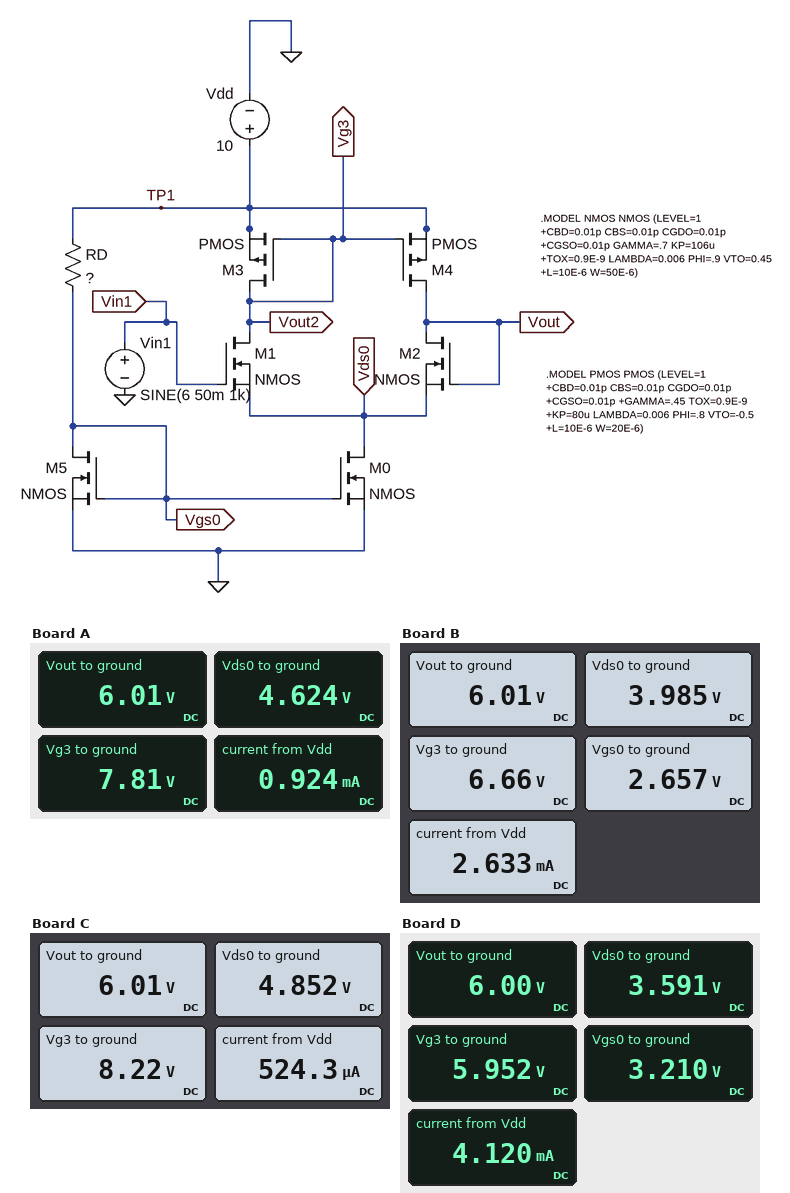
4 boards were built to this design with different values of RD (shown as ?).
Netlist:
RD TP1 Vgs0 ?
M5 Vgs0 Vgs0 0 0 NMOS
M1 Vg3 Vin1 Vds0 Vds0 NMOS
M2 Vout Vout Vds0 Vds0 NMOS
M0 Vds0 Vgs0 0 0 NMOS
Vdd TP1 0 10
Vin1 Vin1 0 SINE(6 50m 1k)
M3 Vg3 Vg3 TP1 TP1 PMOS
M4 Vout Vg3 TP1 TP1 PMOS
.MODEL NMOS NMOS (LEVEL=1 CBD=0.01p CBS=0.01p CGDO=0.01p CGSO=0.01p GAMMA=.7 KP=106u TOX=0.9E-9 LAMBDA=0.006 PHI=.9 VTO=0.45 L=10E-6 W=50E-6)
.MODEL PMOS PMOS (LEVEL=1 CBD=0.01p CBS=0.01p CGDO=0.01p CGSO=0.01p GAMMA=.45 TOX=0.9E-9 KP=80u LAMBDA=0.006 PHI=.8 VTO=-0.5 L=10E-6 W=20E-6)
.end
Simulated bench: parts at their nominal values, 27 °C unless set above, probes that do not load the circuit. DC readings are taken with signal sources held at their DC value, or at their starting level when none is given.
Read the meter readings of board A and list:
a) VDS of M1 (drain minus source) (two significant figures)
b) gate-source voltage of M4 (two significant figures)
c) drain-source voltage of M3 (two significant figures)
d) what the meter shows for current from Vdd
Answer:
3.2 V
-2.2 V
-2.2 V
0.924 mA
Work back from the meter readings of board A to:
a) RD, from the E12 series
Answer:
18 kΩ
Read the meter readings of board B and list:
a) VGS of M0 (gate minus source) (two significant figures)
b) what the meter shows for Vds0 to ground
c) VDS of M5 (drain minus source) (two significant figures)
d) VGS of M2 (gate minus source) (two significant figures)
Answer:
2.7 V
3.985 V
2.7 V
2.0 V
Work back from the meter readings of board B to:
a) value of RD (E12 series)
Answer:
5.6 kΩ
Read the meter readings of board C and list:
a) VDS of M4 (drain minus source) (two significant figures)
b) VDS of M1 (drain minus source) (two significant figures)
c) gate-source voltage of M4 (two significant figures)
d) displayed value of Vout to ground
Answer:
-4.0 V
3.4 V
-1.8 V
6.01 V
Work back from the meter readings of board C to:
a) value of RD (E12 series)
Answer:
33 kΩ
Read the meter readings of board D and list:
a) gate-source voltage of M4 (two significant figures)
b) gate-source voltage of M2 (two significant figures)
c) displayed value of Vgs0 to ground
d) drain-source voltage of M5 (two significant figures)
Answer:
-4.0 V
2.4 V
3.210 V
3.2 V
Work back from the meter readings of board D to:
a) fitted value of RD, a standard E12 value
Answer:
3.3 kΩ
